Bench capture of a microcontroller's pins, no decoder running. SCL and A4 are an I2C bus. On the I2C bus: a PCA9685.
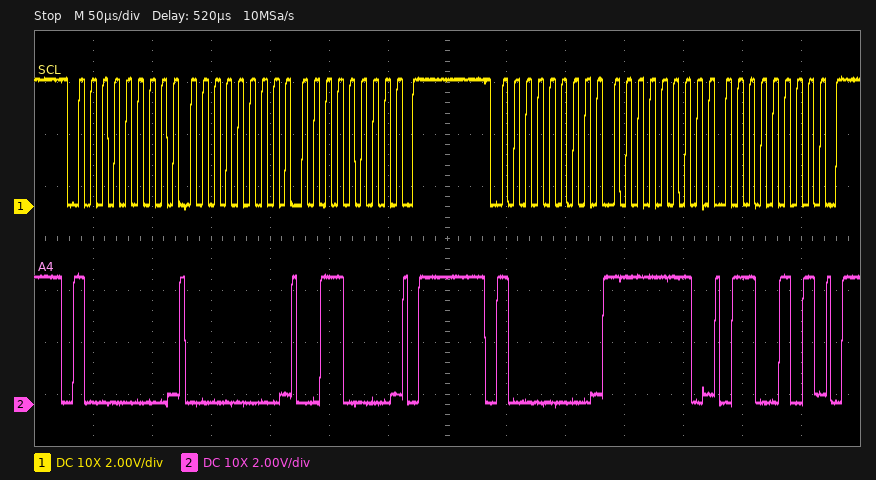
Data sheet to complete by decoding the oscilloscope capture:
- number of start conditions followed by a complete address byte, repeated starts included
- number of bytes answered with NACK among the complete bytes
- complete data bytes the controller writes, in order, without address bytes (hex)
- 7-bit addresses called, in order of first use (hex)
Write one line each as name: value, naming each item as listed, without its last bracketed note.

number of start conditions followed by a complete address byte, repeated starts included: 2
number of bytes answered with NACK among the complete bytes: 0
complete data bytes the controller writes, in order, without address bytes: 00 30 FE 65
7-bit addresses called, in order of first use: 0x40
